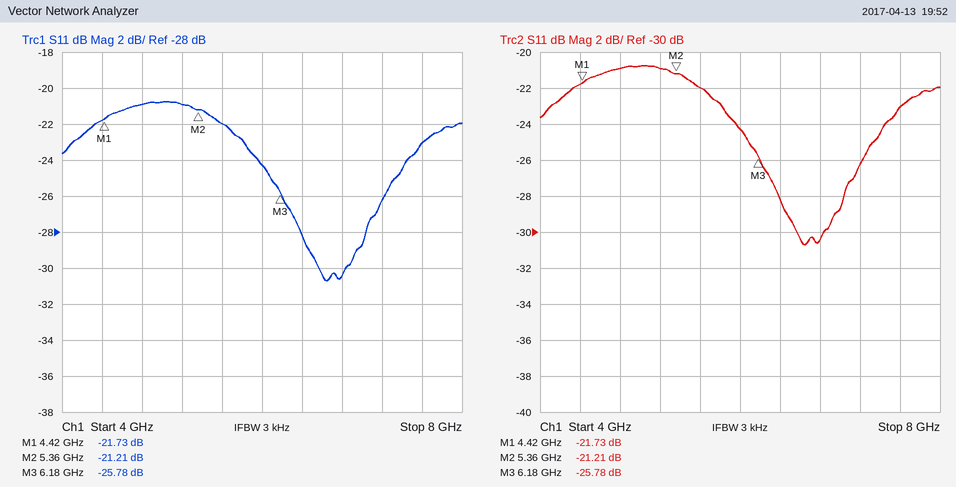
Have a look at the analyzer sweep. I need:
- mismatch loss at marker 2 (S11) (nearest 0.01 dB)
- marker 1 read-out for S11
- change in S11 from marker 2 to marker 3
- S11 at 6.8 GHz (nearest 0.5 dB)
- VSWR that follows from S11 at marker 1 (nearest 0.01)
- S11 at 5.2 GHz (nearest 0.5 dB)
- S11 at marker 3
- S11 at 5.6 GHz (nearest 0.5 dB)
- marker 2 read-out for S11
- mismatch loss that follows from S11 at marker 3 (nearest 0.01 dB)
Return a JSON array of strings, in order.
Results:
["0.03 dB", "-21.73 dB", "-4.57 dB", "-30.5 dB", "1.18", "-21.0 dB", "-25.78 dB", "-22.0 dB", "-21.21 dB", "0.01 dB"]
